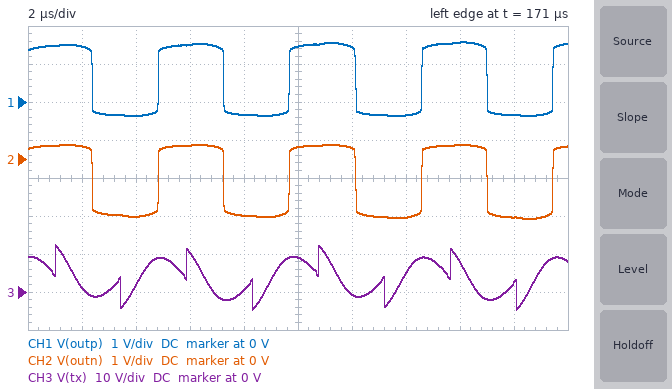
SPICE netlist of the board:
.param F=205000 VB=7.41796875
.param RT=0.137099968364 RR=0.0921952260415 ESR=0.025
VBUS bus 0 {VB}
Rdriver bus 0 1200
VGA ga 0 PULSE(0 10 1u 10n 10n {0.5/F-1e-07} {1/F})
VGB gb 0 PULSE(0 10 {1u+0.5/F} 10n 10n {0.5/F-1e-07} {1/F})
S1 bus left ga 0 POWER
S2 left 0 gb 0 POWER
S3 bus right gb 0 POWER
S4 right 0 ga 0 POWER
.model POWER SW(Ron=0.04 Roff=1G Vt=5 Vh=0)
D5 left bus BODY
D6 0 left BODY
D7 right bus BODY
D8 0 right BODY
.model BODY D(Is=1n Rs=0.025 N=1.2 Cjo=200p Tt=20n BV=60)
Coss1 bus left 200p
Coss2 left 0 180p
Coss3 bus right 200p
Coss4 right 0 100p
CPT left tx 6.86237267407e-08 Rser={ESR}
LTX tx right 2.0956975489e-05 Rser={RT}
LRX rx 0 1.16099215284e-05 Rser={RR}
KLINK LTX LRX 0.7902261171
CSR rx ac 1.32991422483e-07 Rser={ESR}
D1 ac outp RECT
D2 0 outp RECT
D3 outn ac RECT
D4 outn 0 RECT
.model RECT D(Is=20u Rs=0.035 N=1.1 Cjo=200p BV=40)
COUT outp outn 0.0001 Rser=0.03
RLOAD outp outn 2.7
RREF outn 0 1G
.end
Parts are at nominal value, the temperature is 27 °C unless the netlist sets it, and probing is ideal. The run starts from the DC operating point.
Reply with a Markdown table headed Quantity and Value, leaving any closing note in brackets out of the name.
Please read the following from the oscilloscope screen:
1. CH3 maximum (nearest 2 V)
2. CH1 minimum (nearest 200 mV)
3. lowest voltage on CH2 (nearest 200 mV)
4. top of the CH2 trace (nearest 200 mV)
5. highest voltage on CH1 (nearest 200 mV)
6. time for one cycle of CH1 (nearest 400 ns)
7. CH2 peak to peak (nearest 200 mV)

| Quantity | Value |
|---|---|
| CH3 maximum | 12 V |
| CH1 minimum | -400 mV |
| lowest voltage on CH2 | -1.6 V |
| top of the CH2 trace | 400 mV |
| highest voltage on CH1 | 1.6 V |
| time for one cycle of CH1 | 4.8 µs |
| CH2 peak to peak | 2.0 V |
